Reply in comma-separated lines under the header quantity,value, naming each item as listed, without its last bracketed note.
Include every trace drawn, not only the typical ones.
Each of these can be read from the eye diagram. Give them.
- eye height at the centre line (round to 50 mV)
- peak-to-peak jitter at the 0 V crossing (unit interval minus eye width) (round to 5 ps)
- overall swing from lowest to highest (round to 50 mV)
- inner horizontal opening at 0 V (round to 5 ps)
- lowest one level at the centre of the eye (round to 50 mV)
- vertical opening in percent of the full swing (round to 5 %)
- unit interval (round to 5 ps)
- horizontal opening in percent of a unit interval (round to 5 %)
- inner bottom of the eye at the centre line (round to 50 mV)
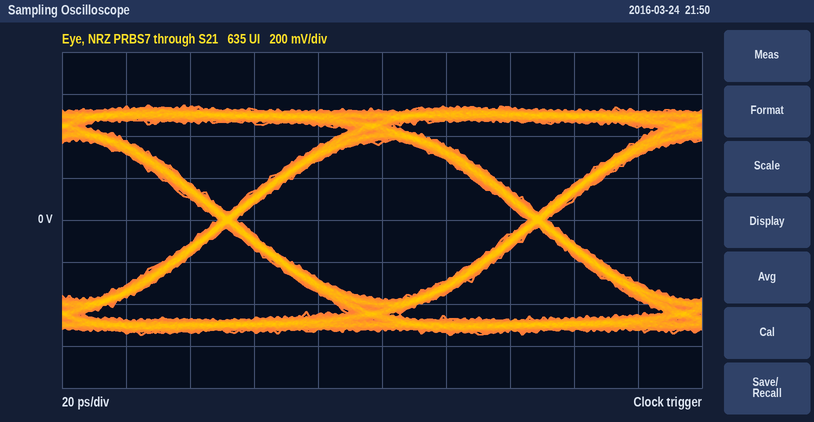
quantity,value
eye height at the centre line,750 mV
peak-to-peak jitter at the 0 V crossing (unit interval minus eye width),5 ps
overall swing from lowest to highest,1.10 V
inner horizontal opening at 0 V,90 ps
lowest one level at the centre of the eye,350 mV
vertical opening in percent of the full swing,70 %
unit interval,95 ps
horizontal opening in percent of a unit interval,95 %
inner bottom of the eye at the centre line,-400 mV
